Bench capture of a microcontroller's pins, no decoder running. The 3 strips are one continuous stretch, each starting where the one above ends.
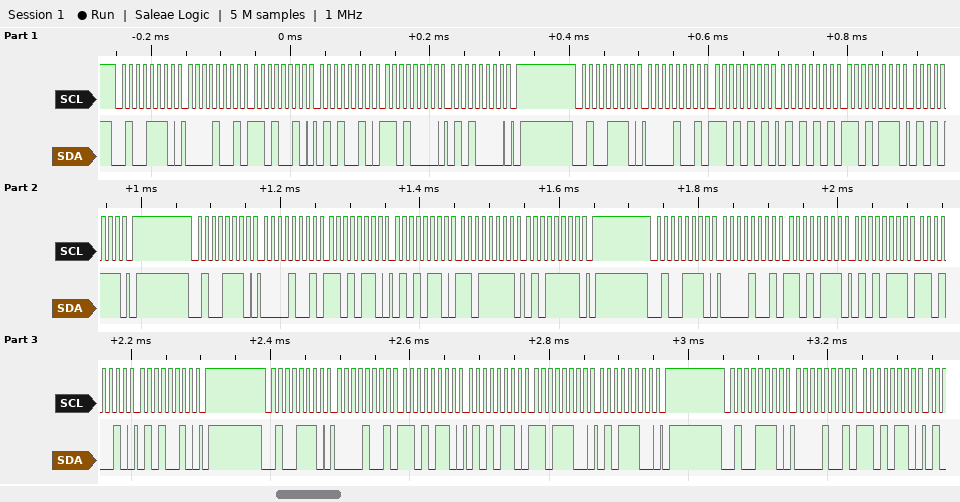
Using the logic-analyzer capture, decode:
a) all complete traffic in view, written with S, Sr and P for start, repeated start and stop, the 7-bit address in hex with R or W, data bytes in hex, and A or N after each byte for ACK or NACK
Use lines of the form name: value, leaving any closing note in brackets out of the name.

all complete traffic in view, written with S, Sr and P for start, repeated start and stop, the 7-bit address in hex with R or W, data bytes in hex, and A or N after each byte for ACK or NACK: S 27W A 09 A D2 A 52 A D0 A 50 A P S 27W A 09 A D5 A 55 A D7 A 57 A P S 27W A 09 A D6 A 56 A DF A 5F A P S 27W A 09 A D7 A 57 A D2 A 52 A P S 27W A 09 A D6 A 56 A DC A 5C A P S 27W A 09 A D6 A
